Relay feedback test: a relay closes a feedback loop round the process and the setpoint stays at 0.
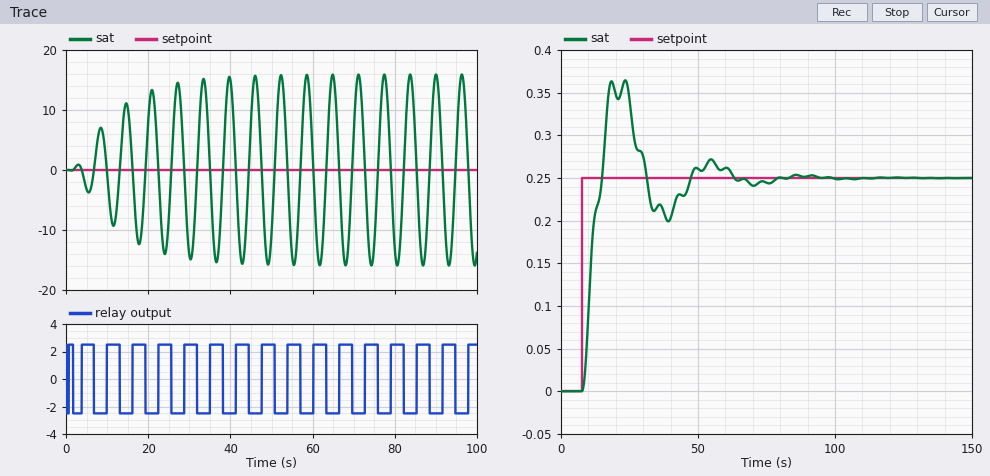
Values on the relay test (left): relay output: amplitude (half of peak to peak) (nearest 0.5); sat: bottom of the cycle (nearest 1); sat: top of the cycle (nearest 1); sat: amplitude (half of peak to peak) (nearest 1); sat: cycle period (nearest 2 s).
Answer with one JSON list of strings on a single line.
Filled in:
["2.5", "-16", "16", "16", "6 s"]
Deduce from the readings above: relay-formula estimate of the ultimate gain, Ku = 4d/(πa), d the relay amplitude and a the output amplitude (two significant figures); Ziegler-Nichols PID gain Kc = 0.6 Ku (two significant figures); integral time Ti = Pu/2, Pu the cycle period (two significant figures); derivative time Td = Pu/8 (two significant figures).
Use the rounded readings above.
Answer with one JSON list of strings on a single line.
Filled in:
["0.20", "0.12", "3.0 s", "0.75 s"]
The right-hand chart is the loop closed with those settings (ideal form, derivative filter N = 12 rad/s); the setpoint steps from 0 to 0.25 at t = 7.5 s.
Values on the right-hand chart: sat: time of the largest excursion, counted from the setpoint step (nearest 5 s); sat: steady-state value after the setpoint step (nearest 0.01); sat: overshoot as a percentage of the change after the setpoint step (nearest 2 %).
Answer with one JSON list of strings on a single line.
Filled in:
["15 s", "0.25", "46 %"]
